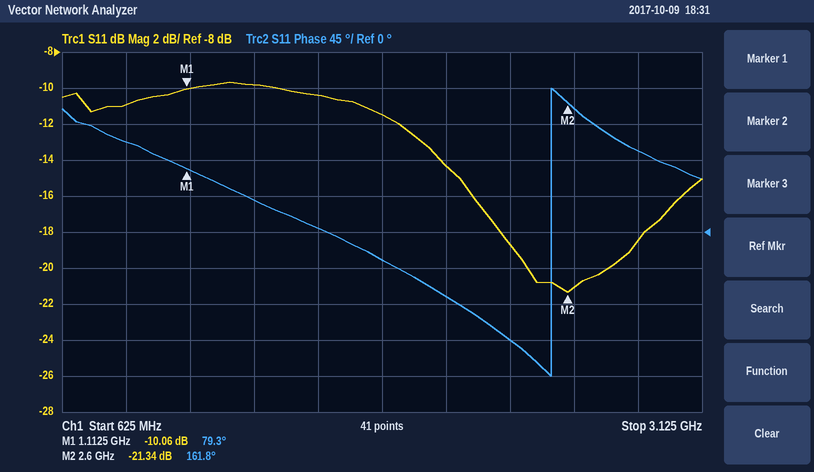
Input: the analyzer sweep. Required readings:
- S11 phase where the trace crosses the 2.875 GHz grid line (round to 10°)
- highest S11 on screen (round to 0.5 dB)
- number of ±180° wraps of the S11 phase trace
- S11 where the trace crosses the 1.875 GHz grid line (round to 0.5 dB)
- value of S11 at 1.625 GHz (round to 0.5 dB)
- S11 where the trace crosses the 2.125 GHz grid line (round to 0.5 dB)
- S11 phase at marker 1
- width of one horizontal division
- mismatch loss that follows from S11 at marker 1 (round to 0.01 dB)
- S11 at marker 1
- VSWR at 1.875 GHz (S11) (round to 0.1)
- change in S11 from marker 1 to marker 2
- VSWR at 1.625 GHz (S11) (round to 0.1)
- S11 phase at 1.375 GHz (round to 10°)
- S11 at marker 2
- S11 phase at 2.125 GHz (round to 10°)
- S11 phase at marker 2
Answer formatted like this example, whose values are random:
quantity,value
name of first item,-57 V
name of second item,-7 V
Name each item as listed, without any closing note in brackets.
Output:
quantity,value
S11 phase where the trace crosses the 2.875 GHz grid line,100°
highest S11 on screen,-9.5 dB
number of ±180° wraps of the S11 phase trace,1
S11 where the trace crosses the 1.875 GHz grid line,-11.5 dB
value of S11 at 1.625 GHz,-10.5 dB
S11 where the trace crosses the 2.125 GHz grid line,-14.5 dB
S11 phase at marker 1,79.3°
width of one horizontal division,250 MHz
mismatch loss that follows from S11 at marker 1,0.45 dB
S11 at marker 1,-10.06 dB
VSWR at 1.875 GHz (S11),1.7
change in S11 from marker 1 to marker 2,-11.28 dB
VSWR at 1.625 GHz (S11),1.9
S11 phase at 1.375 GHz,40°
S11 at marker 2,-21.34 dB
S11 phase at 2.125 GHz,-80°
S11 phase at marker 2,161.8°
